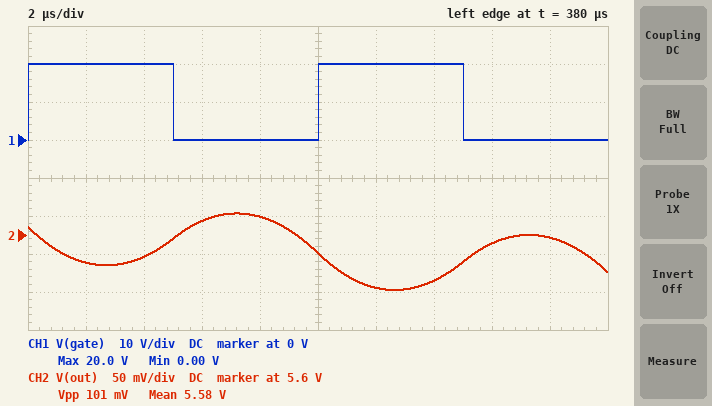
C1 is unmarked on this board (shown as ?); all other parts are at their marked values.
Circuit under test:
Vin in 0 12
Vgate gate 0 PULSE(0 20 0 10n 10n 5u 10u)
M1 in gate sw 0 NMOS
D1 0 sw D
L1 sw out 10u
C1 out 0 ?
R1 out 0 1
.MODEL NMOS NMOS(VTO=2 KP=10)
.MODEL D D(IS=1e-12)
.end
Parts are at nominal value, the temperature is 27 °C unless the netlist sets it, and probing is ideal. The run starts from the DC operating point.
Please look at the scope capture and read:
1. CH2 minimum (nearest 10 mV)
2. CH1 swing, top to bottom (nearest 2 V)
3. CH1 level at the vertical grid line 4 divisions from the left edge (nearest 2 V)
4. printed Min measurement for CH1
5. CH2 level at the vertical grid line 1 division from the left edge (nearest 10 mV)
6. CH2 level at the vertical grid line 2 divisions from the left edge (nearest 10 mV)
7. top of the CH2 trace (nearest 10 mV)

5.53 V
20 V
0 V
0.00 V
5.56 V
5.57 V
5.63 V
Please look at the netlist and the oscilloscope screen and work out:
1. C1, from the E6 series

47 µF
